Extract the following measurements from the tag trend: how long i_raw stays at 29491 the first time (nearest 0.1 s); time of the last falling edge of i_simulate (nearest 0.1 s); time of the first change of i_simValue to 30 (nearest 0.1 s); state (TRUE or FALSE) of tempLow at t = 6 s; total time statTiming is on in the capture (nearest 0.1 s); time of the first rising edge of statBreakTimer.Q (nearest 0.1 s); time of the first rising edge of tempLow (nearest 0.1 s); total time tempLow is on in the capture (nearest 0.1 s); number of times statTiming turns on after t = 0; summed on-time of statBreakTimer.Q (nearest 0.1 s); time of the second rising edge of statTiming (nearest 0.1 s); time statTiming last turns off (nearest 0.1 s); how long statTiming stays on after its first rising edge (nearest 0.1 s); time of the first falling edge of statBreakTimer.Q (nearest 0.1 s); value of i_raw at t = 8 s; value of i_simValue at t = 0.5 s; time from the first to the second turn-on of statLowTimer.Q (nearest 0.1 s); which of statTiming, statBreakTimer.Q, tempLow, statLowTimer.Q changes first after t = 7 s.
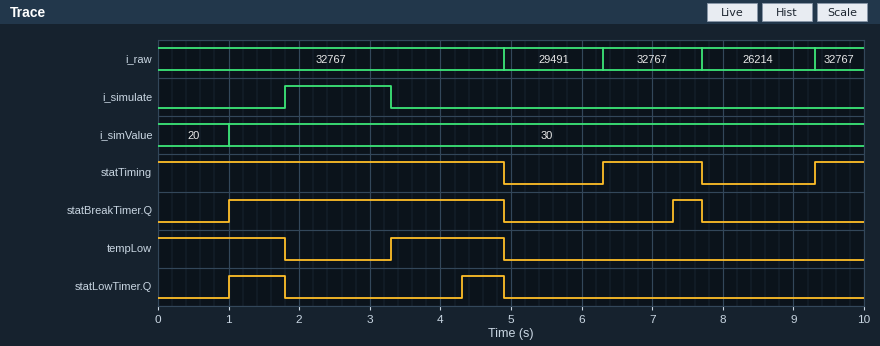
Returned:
1.4 s
3.3 s
1.0 s
FALSE
7.0 s
1.0 s
3.3 s
3.4 s
2
4.3 s
9.3 s
7.7 s
1.4 s
4.9 s
26214
20
3.3 s
statBreakTimer.Q
